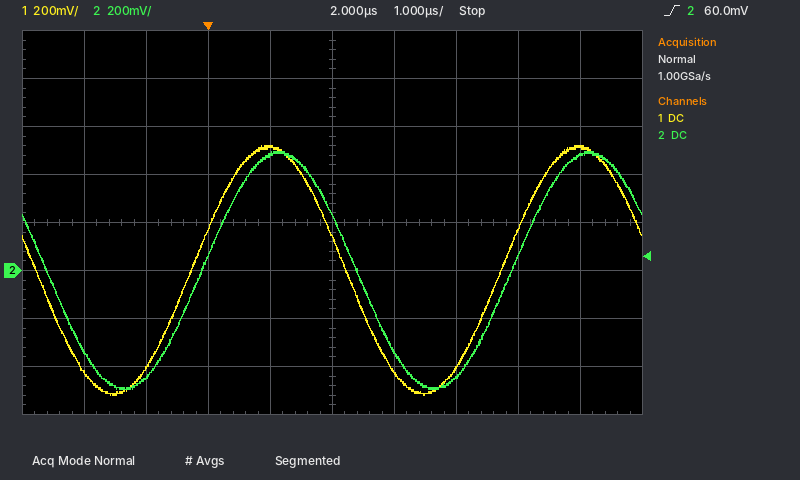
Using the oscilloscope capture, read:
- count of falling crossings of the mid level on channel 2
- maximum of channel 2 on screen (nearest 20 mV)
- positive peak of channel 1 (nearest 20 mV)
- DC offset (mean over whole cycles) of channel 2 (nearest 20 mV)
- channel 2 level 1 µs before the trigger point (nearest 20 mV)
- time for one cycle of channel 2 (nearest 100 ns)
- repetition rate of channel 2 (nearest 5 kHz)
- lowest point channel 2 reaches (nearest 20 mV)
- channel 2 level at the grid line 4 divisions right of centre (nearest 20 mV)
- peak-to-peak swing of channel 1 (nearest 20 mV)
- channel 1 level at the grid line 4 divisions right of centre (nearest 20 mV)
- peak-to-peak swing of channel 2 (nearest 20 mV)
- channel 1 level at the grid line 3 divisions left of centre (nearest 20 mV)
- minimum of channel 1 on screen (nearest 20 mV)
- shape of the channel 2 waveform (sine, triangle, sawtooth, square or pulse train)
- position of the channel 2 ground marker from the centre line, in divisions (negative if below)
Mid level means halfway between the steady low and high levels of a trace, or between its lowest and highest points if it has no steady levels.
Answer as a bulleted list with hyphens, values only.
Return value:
- 2
- 500 mV
- 520 mV
- 0 mV
- -440 mV
- 5.0 µs
- 200 kHz
- -500 mV
- 480 mV
- 1.04 V
- 520 mV
- 1.00 V
- -400 mV
- -520 mV
- sine
- -1.0 div
